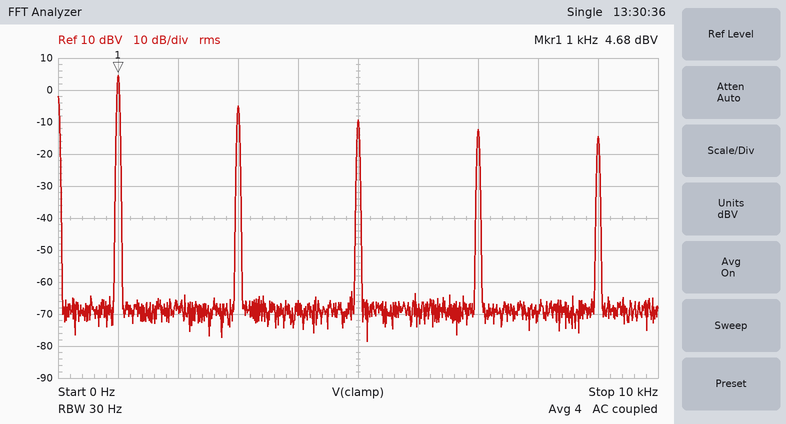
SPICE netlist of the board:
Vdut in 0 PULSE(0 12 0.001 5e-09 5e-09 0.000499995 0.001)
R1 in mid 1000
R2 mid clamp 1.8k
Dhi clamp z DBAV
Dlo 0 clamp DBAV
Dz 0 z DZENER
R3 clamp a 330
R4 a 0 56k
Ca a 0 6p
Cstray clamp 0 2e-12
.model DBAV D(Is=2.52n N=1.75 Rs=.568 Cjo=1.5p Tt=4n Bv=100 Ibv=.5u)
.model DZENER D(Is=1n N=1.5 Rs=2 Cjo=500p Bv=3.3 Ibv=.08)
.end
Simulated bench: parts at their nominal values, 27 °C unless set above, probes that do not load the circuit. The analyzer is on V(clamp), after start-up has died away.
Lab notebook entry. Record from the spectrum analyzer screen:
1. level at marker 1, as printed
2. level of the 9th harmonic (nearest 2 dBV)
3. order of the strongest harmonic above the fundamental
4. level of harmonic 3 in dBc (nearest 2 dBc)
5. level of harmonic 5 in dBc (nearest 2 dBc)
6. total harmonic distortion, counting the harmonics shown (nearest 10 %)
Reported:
4.68 dBV
-14 dBV
3
-10 dBc
-14 dBc
40 %
